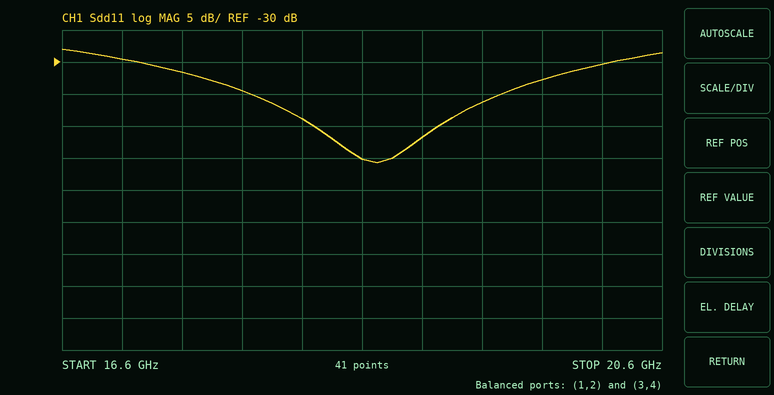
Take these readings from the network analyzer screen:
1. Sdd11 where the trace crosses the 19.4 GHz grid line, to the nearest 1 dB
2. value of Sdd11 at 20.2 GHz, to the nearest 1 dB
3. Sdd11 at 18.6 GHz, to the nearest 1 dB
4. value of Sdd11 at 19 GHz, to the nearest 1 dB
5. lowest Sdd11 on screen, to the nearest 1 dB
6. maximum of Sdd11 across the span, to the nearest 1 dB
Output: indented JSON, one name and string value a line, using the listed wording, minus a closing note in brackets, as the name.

{
  "Sdd11 where the trace crosses the 19.4 GHz grid line, to the nearest 1 dB": "-36 dB",
  "value of Sdd11 at 20.2 GHz, to the nearest 1 dB": "-30 dB",
  "Sdd11 at 18.6 GHz, to the nearest 1 dB": "-45 dB",
  "value of Sdd11 at 19 GHz, to the nearest 1 dB": "-42 dB",
  "lowest Sdd11 on screen, to the nearest 1 dB": "-46 dB",
  "maximum of Sdd11 across the span, to the nearest 1 dB": "-28 dB"
}
